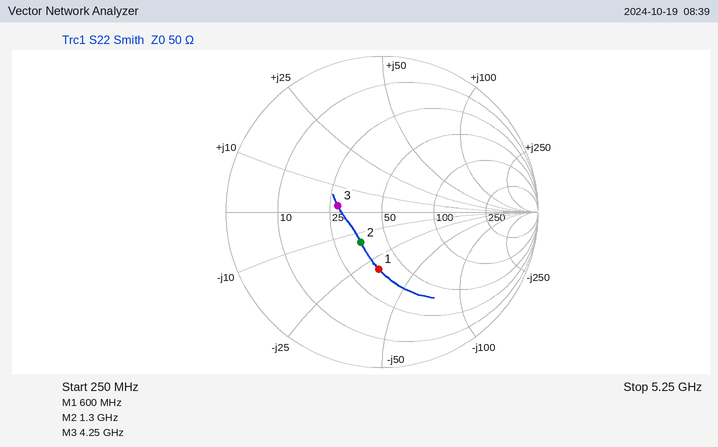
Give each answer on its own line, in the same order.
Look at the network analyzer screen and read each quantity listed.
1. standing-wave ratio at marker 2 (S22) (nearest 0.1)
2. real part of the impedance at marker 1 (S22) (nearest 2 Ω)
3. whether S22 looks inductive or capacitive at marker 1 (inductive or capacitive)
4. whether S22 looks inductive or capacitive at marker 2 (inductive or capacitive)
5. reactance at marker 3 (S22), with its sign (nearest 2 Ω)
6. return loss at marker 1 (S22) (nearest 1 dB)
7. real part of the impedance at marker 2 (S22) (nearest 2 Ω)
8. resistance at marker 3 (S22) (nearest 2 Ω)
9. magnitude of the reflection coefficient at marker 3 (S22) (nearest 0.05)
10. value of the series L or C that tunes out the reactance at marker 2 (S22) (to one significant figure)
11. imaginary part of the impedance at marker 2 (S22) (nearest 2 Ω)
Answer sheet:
1.6
36 Ω
capacitive
capacitive
+2 Ω
9 dB
36 Ω
28 Ω
0.30
2 nH
-14 Ω
